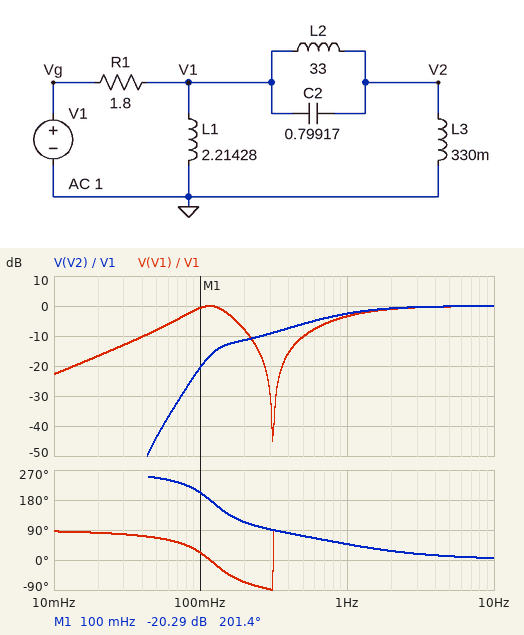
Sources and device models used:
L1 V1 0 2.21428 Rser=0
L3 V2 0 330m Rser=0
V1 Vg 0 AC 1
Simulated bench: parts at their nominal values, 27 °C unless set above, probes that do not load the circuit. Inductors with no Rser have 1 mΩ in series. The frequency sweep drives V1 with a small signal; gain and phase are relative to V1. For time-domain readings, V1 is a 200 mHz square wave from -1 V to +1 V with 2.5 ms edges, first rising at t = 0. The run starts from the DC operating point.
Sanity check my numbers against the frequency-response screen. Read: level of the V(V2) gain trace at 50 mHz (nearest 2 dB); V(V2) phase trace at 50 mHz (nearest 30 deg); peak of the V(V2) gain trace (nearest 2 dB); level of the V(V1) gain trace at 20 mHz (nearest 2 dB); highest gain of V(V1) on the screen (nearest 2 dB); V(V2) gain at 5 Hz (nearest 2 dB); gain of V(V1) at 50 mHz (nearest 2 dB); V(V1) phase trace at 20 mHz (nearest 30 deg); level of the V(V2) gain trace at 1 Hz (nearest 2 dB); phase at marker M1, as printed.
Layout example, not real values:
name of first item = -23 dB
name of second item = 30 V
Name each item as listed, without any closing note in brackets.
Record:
level of the V(V2) gain trace at 50 mHz = -44 dB
V(V2) phase trace at 50 mHz = 240 deg
peak of the V(V2) gain trace = 0 dB
level of the V(V1) gain trace at 20 mHz = -16 dB
highest gain of V(V1) on the screen = 0 dB
V(V2) gain at 5 Hz = 0 dB
gain of V(V1) at 50 mHz = -8 dB
V(V1) phase trace at 20 mHz = 90 deg
level of the V(V2) gain trace at 1 Hz = -2 dB
phase at marker M1, as printed = 201.4 deg
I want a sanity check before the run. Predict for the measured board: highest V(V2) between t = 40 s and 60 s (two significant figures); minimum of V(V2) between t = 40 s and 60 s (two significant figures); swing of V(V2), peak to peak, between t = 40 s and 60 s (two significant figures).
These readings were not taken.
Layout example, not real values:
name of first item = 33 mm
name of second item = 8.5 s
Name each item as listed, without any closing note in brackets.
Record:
highest V(V2) between t = 40 s and 60 s = 2.1 V
minimum of V(V2) between t = 40 s and 60 s = -2.1 V
swing of V(V2), peak to peak, between t = 40 s and 60 s = 4.2 V
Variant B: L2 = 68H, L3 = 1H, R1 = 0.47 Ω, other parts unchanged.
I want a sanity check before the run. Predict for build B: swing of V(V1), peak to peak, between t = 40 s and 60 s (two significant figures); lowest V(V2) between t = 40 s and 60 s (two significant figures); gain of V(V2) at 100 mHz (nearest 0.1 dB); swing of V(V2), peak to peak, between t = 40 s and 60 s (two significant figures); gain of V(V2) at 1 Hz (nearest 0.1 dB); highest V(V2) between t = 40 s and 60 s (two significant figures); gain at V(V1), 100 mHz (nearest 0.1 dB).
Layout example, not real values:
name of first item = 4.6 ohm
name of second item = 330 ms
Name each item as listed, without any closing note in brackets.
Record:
swing of V(V1), peak to peak, between t = 40 s and 60 s = 3.3 V
lowest V(V2) between t = 40 s and 60 s = -3.7 V
gain of V(V2) at 100 mHz = -7.3 dB
swing of V(V2), peak to peak, between t = 40 s and 60 s = 7.4 V
gain of V(V2) at 1 Hz = 0.2 dB
highest V(V2) between t = 40 s and 60 s = 3.7 V
gain at V(V1), 100 mHz = 0 dB
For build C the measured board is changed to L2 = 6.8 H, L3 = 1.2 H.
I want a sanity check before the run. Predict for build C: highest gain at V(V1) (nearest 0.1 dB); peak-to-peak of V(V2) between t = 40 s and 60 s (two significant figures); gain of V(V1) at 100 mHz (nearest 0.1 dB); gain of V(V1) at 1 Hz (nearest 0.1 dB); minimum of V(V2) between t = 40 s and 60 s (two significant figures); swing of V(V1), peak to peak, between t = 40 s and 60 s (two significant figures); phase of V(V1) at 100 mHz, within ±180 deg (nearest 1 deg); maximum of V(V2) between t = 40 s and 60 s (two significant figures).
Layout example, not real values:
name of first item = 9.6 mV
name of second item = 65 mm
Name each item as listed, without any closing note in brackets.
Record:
highest gain at V(V1) = 0 dB
peak-to-peak of V(V2) between t = 40 s and 60 s = 4.8 V
gain of V(V1) at 100 mHz = -1.7 dB
gain of V(V1) at 1 Hz = -0.6 dB
minimum of V(V2) between t = 40 s and 60 s = -2.4 V
swing of V(V1), peak to peak, between t = 40 s and 60 s = 3.4 V
phase of V(V1) at 100 mHz, within ±180 deg = 35 deg
maximum of V(V2) between t = 40 s and 60 s = 2.4 V
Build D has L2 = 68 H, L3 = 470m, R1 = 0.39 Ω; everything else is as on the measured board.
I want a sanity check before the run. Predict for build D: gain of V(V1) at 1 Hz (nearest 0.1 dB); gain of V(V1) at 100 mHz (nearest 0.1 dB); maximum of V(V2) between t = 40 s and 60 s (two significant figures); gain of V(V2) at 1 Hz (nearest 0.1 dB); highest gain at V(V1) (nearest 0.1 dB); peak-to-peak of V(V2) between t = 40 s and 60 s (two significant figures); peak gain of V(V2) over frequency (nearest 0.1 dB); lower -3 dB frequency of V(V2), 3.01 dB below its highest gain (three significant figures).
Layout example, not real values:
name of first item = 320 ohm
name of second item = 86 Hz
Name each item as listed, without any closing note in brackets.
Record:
gain of V(V1) at 1 Hz = -0.1 dB
gain of V(V1) at 100 mHz = 0 dB
maximum of V(V2) between t = 40 s and 60 s = 2.2 V
gain of V(V2) at 1 Hz = 0.5 dB
highest gain at V(V1) = 0 dB
peak-to-peak of V(V2) between t = 40 s and 60 s = 4.3 V
peak gain of V(V2) over frequency = 6.0 dB
lower -3 dB frequency of V(V2), 3.01 dB below its highest gain = 217 mHz
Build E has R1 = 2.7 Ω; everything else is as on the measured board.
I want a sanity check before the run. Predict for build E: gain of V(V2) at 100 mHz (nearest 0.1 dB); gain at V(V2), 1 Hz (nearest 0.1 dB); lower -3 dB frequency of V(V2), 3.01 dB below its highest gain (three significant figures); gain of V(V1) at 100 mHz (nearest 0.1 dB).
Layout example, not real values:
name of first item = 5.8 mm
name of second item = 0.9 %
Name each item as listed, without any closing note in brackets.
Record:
gain of V(V2) at 100 mHz = -21.0 dB
gain at V(V2), 1 Hz = -4.8 dB
lower -3 dB frequency of V(V2), 3.01 dB below its highest gain = 1.42 Hz
gain of V(V1) at 100 mHz = -1.3 dB
